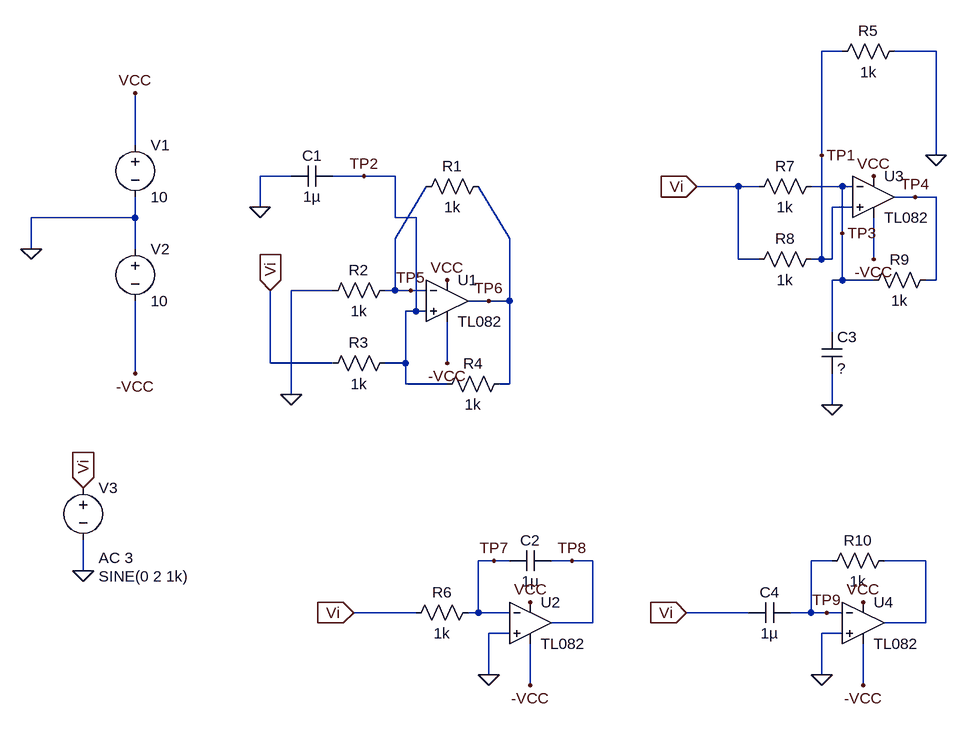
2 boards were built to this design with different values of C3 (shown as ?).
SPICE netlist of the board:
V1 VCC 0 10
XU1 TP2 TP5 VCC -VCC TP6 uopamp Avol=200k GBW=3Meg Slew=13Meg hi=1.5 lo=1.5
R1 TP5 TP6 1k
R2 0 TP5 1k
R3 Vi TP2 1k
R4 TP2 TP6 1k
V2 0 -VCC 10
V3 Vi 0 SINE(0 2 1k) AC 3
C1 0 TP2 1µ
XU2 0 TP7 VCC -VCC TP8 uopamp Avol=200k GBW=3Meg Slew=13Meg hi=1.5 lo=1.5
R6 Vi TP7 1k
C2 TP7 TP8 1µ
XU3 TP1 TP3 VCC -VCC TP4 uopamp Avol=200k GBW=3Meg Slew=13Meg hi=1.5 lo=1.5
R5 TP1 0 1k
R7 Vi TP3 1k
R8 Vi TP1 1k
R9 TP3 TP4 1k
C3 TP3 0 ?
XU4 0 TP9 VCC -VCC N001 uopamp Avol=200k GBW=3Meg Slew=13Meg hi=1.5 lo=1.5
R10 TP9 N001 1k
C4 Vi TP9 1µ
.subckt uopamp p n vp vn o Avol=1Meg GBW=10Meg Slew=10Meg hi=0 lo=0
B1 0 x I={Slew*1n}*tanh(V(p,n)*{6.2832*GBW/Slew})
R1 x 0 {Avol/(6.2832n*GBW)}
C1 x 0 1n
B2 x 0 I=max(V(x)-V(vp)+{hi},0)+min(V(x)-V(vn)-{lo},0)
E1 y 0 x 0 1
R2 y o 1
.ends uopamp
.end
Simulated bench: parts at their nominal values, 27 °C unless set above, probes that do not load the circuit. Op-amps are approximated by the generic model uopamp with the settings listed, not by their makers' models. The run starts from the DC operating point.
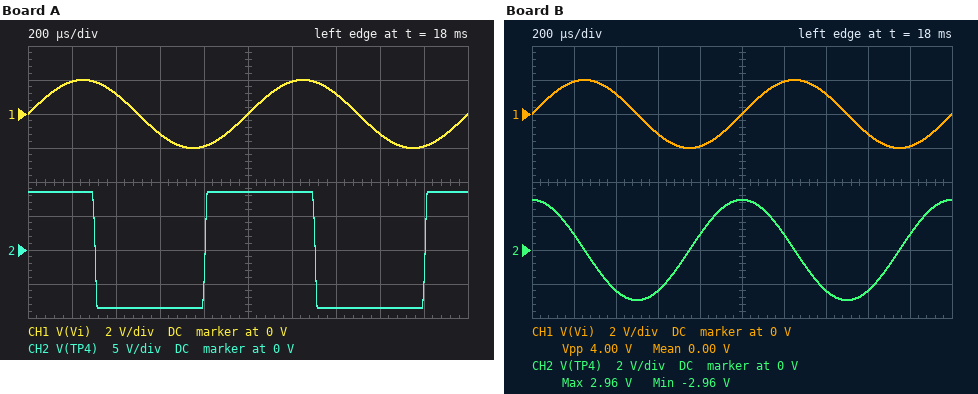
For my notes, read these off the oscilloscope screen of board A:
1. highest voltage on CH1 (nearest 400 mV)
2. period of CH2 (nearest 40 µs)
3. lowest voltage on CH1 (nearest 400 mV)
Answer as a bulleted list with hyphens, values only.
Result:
- 2.0 V
- 1.00 ms
- -2.0 V
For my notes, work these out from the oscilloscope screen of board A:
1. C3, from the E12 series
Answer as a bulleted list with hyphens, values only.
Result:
- 2.2 µF
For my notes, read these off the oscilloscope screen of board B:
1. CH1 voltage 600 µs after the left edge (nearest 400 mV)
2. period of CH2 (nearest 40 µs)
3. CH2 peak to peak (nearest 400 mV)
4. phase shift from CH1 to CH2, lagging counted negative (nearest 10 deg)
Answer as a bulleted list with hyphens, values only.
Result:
- -1.2 V
- 1.00 ms
- 6.0 V
- 90 deg
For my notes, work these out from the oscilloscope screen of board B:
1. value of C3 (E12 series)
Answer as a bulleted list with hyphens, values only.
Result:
- 470 nF
